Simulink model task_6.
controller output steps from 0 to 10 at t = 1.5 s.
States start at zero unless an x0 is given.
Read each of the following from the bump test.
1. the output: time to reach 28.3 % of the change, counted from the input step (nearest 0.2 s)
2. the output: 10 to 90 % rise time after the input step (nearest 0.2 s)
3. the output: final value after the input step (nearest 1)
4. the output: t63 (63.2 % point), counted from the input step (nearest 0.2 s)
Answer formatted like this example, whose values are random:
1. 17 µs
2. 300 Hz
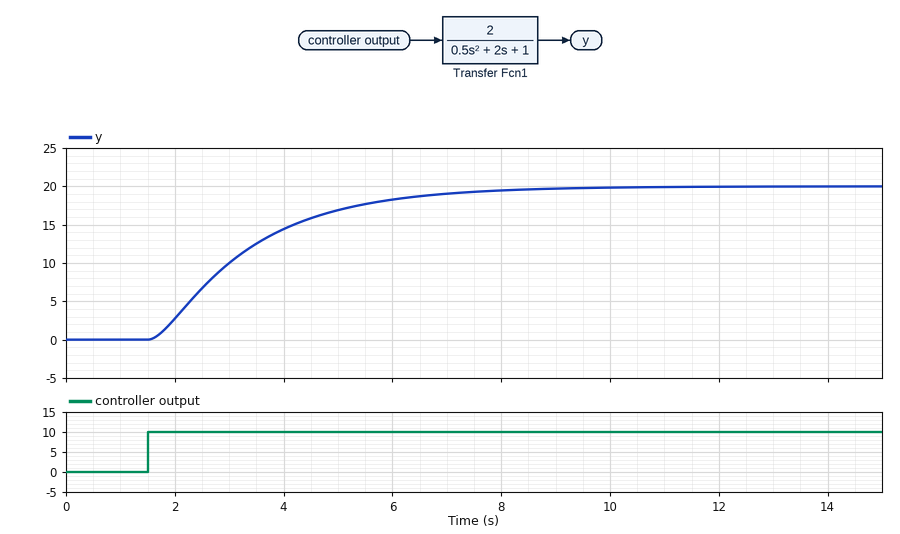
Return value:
1. 0.8 s
2. 3.8 s
3. 20
4. 2.0 s
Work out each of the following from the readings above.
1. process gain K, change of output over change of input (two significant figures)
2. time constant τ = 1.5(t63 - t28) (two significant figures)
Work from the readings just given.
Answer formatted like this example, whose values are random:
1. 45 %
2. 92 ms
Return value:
1. 2.0
2. 1.8 s
